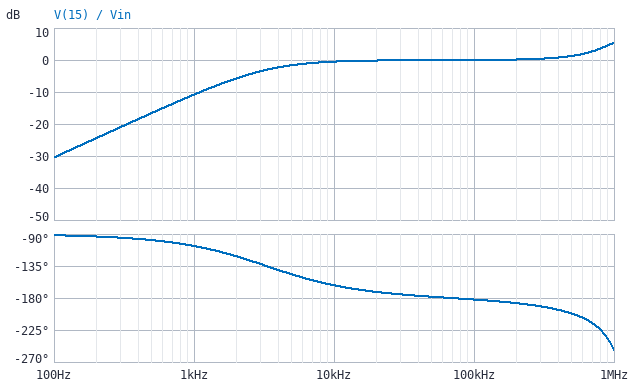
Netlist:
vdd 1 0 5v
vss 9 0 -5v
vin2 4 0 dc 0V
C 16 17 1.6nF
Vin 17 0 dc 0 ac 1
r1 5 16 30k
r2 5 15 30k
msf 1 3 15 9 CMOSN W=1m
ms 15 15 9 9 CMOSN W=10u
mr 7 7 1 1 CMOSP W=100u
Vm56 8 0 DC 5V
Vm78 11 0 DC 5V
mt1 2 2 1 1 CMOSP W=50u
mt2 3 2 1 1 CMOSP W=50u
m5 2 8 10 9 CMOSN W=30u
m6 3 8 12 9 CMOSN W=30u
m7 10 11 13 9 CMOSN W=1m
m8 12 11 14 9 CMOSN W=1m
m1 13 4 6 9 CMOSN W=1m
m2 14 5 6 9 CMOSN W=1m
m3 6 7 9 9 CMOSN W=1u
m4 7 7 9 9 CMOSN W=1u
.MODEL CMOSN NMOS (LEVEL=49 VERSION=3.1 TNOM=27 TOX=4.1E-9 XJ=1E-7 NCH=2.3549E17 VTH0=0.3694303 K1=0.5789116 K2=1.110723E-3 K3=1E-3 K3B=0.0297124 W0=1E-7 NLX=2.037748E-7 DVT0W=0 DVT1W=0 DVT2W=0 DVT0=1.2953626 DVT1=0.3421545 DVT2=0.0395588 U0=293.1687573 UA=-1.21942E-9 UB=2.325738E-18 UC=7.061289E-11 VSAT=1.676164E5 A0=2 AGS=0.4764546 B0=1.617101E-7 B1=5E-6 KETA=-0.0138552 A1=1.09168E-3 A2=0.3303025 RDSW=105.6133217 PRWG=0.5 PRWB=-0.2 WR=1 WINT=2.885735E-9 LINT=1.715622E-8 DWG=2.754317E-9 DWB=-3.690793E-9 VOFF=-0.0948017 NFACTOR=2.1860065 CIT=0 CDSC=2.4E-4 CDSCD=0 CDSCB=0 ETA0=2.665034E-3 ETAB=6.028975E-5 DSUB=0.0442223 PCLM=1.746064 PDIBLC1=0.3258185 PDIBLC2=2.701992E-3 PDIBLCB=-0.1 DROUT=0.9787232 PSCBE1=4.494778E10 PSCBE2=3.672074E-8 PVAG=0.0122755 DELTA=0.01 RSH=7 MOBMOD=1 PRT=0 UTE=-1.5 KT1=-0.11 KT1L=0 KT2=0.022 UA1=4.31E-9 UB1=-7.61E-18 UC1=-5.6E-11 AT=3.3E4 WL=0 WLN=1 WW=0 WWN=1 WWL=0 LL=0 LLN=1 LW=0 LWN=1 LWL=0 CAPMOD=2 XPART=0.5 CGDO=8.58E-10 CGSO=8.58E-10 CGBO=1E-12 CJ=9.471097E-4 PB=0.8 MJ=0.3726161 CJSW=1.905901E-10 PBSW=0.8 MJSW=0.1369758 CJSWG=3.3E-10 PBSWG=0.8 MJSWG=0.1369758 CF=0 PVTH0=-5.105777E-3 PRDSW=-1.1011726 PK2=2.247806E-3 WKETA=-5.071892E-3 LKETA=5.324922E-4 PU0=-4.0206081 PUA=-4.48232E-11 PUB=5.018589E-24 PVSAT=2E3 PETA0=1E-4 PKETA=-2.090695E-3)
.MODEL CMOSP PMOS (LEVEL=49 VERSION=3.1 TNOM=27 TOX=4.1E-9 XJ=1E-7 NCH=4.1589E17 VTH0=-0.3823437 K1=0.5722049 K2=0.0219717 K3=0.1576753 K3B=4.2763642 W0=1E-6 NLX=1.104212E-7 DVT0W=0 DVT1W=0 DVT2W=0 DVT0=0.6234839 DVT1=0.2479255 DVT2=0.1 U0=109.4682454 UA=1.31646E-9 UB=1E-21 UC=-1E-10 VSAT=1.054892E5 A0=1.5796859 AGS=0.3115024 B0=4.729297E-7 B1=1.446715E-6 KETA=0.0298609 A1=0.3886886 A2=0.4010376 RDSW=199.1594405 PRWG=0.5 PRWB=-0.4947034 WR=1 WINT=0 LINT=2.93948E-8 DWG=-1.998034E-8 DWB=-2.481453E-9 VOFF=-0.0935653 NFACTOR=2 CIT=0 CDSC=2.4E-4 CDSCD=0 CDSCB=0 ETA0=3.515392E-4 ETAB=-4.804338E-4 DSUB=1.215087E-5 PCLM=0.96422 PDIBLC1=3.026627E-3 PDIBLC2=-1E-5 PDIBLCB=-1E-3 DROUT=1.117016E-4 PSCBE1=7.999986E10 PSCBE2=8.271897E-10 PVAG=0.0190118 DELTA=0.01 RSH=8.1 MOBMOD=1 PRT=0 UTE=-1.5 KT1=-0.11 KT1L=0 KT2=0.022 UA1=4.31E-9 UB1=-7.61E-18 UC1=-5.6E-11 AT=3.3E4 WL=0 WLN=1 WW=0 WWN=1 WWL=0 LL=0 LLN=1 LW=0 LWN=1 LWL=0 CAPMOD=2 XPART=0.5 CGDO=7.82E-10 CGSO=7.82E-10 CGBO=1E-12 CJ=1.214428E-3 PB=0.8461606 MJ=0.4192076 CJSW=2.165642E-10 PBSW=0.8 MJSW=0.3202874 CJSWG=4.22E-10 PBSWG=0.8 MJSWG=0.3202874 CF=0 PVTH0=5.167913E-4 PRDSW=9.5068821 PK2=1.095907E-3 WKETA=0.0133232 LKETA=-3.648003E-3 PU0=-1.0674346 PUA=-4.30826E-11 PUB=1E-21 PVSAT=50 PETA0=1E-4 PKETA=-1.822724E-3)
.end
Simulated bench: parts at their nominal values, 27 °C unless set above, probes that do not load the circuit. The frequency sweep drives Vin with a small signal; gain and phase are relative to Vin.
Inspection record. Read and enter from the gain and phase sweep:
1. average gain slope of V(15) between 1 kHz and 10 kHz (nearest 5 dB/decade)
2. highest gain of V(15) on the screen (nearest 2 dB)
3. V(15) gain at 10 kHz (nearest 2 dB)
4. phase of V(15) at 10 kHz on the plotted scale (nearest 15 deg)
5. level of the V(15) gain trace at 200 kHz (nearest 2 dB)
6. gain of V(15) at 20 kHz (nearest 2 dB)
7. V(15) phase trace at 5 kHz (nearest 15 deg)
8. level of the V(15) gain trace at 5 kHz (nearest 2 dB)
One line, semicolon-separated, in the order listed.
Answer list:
10 dB/decade; 6 dB; 0 dB; -165 deg; 0 dB; 0 dB; -150 deg; -2 dB
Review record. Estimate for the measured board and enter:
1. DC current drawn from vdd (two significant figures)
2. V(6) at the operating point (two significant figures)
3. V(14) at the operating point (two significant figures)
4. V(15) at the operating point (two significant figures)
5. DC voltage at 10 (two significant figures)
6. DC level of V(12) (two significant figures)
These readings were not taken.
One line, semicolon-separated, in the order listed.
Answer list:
3.0 mA; -1.1 V; 1.5 V; 4.7 mV; 3.1 V; 1.5 V
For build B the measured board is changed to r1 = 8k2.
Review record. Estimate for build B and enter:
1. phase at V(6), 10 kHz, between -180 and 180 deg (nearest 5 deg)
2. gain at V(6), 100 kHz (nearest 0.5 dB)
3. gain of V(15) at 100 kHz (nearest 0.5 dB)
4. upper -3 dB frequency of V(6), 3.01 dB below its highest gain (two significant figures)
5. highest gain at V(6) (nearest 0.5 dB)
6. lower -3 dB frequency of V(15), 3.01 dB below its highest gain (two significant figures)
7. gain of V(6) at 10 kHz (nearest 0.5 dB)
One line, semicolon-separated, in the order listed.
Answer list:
120 deg; -28.0 dB; 11.0 dB; 2.1 MHz; -8.5 dB; 12 kHz; -51.5 dB
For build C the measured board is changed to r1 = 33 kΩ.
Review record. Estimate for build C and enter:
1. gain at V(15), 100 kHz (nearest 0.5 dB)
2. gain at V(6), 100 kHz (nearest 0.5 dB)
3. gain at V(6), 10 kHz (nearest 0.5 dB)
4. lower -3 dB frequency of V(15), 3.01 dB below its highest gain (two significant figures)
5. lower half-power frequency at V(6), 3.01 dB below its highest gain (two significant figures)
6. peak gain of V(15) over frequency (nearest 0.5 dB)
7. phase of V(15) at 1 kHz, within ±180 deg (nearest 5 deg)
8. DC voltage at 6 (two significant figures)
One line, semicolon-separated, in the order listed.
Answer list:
-1.0 dB; -40.0 dB; -60.0 dB; 710 kHz; 910 kHz; 5.0 dB; -110 deg; -1.1 V
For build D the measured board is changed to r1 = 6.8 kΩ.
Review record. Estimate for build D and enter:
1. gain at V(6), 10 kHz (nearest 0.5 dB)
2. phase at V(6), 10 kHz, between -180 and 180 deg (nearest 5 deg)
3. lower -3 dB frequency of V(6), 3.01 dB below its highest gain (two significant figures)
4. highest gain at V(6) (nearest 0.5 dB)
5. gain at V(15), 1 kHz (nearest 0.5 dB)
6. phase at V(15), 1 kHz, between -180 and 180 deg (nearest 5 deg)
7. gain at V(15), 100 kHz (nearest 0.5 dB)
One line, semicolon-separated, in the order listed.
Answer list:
-50.5 dB; 125 deg; 570 kHz; -8.5 dB; -10.5 dB; -95 deg; 13.0 dB
